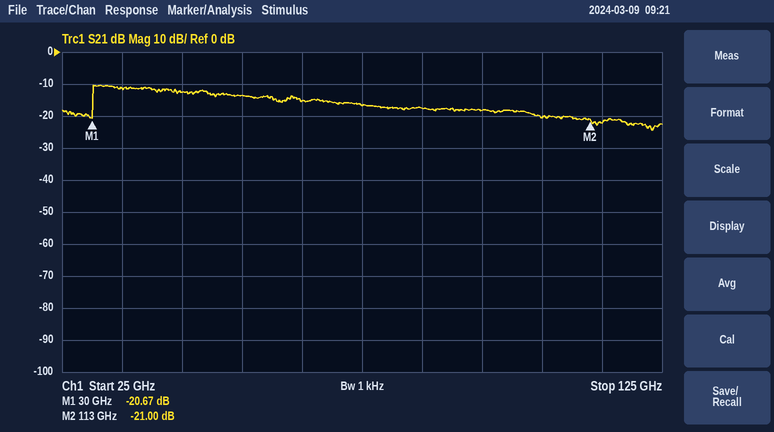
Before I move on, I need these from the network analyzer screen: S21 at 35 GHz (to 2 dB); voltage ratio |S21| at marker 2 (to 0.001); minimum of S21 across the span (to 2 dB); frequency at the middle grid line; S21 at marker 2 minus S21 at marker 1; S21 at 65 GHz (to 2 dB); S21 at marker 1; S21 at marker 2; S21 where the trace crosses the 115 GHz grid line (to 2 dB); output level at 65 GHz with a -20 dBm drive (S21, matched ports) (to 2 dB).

-12 dB
0.089
-24 dB
75 GHz
-0.33 dB
-16 dB
-20.67 dB
-21.00 dB
-22 dB
-36 dBm
